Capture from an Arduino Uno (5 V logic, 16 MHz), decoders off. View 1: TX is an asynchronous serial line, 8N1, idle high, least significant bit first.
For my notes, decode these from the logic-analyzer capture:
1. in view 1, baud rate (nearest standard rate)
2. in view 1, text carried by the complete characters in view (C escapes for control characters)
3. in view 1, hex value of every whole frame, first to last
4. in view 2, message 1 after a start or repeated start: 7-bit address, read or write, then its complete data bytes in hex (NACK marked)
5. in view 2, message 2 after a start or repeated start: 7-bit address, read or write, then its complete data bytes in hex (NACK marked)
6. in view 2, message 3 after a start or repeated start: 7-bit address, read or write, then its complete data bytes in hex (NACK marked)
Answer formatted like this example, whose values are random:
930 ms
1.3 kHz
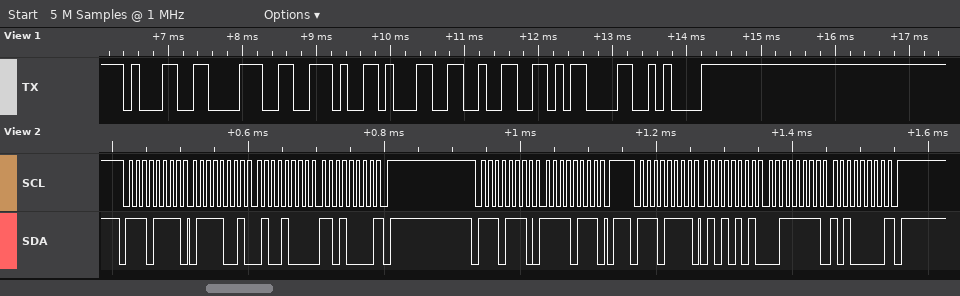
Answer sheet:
9600 baud
"18.12\r\n"
0x31 0x38 0x2E 0x31 0x32 0x0D 0x0A
0x77 read: 79 48 D0 NACK
0x77 write: F7
0x77 read: 55 3F A0 NACK
